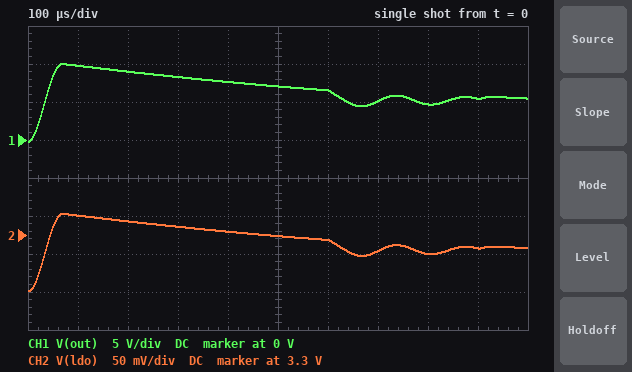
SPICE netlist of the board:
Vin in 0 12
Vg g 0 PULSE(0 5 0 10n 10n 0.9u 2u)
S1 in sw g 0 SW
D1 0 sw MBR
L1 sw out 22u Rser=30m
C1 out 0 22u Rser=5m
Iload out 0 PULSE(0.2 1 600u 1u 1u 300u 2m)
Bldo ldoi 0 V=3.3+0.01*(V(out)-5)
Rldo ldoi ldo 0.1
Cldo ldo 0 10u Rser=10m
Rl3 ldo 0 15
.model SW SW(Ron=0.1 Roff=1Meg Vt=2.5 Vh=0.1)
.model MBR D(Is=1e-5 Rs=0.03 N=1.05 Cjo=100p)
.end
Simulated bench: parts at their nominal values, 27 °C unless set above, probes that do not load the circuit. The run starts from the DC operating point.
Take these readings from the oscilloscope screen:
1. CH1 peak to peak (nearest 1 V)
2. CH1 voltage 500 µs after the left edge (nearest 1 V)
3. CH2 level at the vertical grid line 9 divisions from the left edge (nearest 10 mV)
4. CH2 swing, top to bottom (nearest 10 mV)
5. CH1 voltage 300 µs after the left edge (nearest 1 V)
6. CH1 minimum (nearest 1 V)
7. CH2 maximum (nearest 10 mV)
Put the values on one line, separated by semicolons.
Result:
10 V; 7 V; 3.28 V; 100 mV; 8 V; 0 V; 3.33 V
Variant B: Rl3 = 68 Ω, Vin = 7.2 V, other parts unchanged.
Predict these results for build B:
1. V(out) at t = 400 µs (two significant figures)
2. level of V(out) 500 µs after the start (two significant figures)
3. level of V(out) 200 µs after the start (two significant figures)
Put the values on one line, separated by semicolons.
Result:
3.5 V; 3.0 V; 4.9 V
